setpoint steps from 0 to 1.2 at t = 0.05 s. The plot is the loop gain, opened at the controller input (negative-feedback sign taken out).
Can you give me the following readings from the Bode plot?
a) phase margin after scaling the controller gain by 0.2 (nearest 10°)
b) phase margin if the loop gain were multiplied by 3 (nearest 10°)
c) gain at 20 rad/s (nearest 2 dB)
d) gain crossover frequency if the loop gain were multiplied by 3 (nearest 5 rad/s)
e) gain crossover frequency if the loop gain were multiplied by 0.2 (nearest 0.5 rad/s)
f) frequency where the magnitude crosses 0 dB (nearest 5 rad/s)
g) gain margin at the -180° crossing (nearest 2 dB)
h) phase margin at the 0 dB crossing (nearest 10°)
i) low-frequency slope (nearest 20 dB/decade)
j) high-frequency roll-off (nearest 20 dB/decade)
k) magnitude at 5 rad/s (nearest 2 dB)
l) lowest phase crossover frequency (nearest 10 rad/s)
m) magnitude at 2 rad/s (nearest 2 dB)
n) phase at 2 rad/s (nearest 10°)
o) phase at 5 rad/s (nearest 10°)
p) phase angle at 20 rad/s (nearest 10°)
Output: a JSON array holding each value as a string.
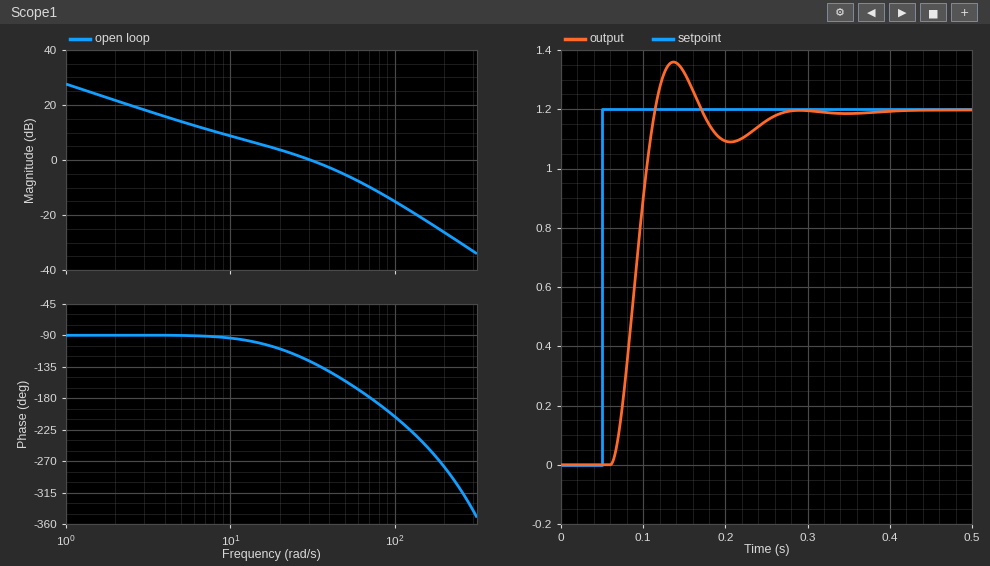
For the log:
["90°", "0°", "4 dB", "70 rad/s", "5.0 rad/s", "30 rad/s", "10 dB", "50°", "-20 dB/decade", "-40 dB/decade", "14 dB", "70 rad/s", "22 dB", "-90°", "-90°", "-110°"]
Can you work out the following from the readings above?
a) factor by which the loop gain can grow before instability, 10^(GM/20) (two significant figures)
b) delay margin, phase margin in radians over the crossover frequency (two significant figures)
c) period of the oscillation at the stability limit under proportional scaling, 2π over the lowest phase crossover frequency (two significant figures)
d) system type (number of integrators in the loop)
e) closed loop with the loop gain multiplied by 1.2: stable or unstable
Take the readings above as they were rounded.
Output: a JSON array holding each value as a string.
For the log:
["3.2", "0.029 s", "0.090 s", "1", "stable"]
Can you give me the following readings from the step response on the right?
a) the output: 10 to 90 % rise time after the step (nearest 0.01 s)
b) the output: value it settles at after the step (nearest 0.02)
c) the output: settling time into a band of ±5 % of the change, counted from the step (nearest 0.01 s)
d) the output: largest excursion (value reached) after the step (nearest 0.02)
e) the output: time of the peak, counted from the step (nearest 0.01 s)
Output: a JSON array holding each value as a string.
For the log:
["0.04 s", "1.20", "0.19 s", "1.36", "0.09 s"]
